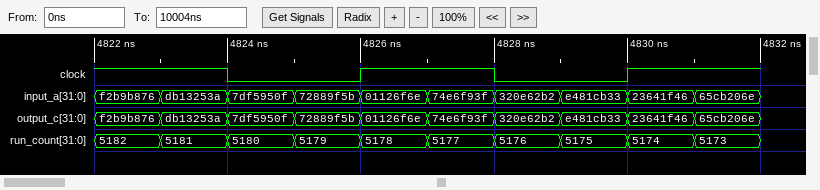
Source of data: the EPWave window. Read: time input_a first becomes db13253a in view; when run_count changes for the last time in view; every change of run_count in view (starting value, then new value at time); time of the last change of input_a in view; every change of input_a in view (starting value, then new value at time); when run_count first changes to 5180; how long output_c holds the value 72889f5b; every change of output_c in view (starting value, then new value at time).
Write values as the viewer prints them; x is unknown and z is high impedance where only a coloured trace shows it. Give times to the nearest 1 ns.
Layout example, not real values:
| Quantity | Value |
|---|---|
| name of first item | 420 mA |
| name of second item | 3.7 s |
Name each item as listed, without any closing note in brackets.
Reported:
| Quantity | Value |
|---|---|
| time input_a first becomes db13253a in view | 4823 ns |
| when run_count changes for the last time in view | 4831 ns |
| every change of run_count in view | 5182, 5181 at 4823 ns, 5180 at 4824 ns, 5179 at 4825 ns, 5178 at 4826 ns, 5177 at 4827 ns, 5176 at 4828 ns, 5175 at 4829 ns, 5174 at 4830 ns, 5173 at 4831 ns |
| time of the last change of input_a in view | 4831 ns |
| every change of input_a in view | f2b9b876, db13253a at 4823 ns, 7df5950f at 4824 ns, 72889f5b at 4825 ns, 01126f6e at 4826 ns, 74e6f93f at 4827 ns, 320e62b2 at 4828 ns, e481cb33 at 4829 ns, 23641f46 at 4830 ns, 65cb206e at 4831 ns |
| when run_count first changes to 5180 | 4824 ns |
| how long output_c holds the value 72889f5b | 1 ns |
| every change of output_c in view | f2b9b876, db13253a at 4823 ns, 7df5950f at 4824 ns, 72889f5b at 4825 ns, 01126f6e at 4826 ns, 74e6f93f at 4827 ns, 320e62b2 at 4828 ns, e481cb33 at 4829 ns, 23641f46 at 4830 ns, 65cb206e at 4831 ns |
